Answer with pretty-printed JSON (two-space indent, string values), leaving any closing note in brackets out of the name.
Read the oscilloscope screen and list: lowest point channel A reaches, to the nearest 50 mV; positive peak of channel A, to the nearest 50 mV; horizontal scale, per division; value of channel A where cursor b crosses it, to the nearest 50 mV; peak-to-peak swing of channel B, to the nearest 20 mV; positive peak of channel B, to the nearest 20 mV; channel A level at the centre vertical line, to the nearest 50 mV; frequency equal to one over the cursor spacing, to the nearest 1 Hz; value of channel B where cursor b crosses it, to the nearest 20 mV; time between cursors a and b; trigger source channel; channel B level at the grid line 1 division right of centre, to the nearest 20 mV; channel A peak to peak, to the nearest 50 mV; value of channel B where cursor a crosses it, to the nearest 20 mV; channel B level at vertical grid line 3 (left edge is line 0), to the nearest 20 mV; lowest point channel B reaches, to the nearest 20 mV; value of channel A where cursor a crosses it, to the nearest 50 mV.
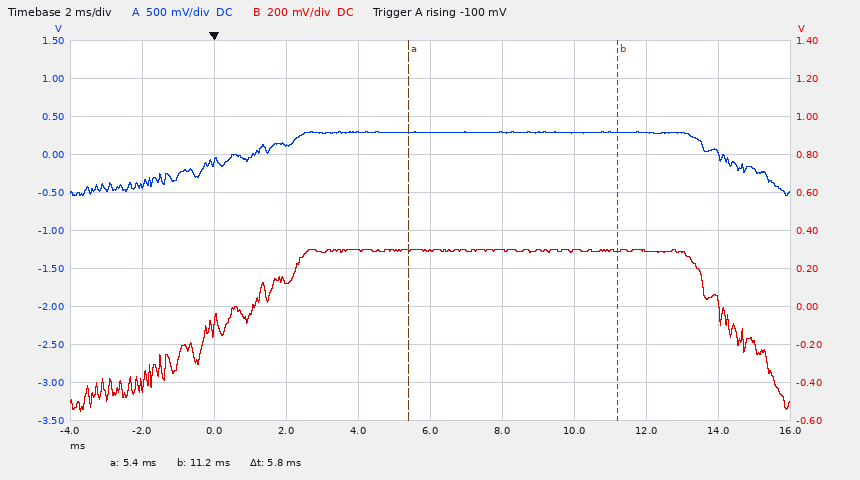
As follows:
{
  "lowest point channel A reaches, to the nearest 50 mV": "-550 mV",
  "positive peak of channel A, to the nearest 50 mV": "300 mV",
  "horizontal scale, per division": "2 ms",
  "value of channel A where cursor b crosses it, to the nearest 50 mV": "300 mV",
  "peak-to-peak swing of channel B, to the nearest 20 mV": "860 mV",
  "positive peak of channel B, to the nearest 20 mV": "300 mV",
  "channel A level at the centre vertical line, to the nearest 50 mV": "300 mV",
  "frequency equal to one over the cursor spacing, to the nearest 1 Hz": "172 Hz",
  "value of channel B where cursor b crosses it, to the nearest 20 mV": "300 mV",
  "time between cursors a and b": "5.8 ms",
  "trigger source channel": "channel A",
  "channel B level at the grid line 1 division right of centre, to the nearest 20 mV": "300 mV",
  "channel A peak to peak, to the nearest 50 mV": "850 mV",
  "value of channel B where cursor a crosses it, to the nearest 20 mV": "300 mV",
  "channel B level at vertical grid line 3 (left edge is line 0), to the nearest 20 mV": "140 mV",
  "lowest point channel B reaches, to the nearest 20 mV": "-560 mV",
  "value of channel A where cursor a crosses it, to the nearest 50 mV": "300 mV"
}
